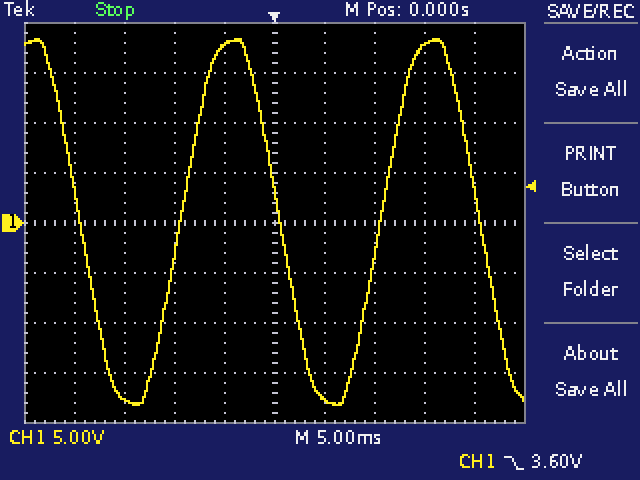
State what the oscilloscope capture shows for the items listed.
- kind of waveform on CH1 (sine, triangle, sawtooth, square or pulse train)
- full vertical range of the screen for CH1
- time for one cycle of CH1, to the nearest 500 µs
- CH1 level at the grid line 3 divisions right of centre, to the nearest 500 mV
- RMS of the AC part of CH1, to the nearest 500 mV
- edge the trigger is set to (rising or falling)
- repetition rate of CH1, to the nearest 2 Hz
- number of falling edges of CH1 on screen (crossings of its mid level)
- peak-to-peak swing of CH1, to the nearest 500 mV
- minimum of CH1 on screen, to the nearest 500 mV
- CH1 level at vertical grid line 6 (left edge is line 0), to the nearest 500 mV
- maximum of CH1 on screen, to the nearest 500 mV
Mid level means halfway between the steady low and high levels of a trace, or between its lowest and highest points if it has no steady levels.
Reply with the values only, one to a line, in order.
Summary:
sine
40 V
20.0 ms
17.5 V
13.0 V
falling
50 Hz
3
36.5 V
-18.0 V
-17.5 V
18.5 V
